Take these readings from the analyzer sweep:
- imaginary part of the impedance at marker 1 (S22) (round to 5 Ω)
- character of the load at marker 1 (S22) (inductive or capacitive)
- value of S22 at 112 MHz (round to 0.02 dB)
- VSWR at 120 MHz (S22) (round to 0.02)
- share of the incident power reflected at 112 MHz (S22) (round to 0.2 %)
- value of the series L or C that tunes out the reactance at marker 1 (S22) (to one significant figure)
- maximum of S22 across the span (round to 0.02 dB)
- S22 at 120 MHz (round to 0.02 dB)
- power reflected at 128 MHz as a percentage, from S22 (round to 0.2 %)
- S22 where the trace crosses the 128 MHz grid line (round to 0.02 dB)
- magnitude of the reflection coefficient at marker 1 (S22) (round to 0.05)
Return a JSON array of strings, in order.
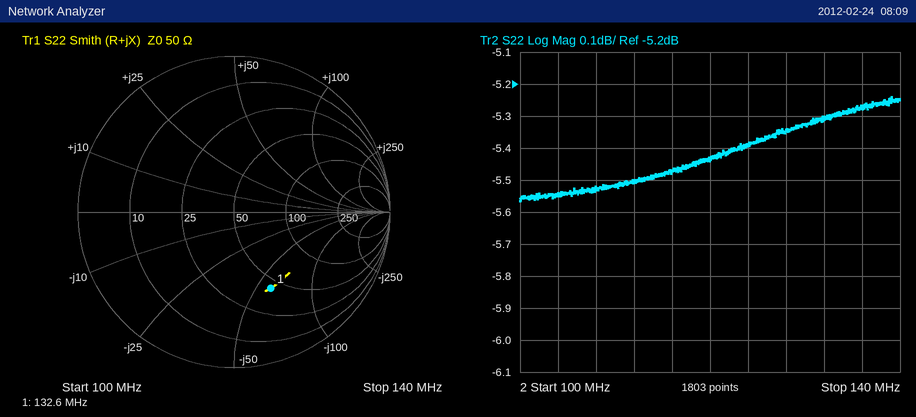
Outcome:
["-60 Ω", "capacitive", "-5.50 dB", "3.30", "28.2 %", "70 nH", "-5.24 dB", "-5.44 dB", "29.2 %", "-5.34 dB", "0.55"]
